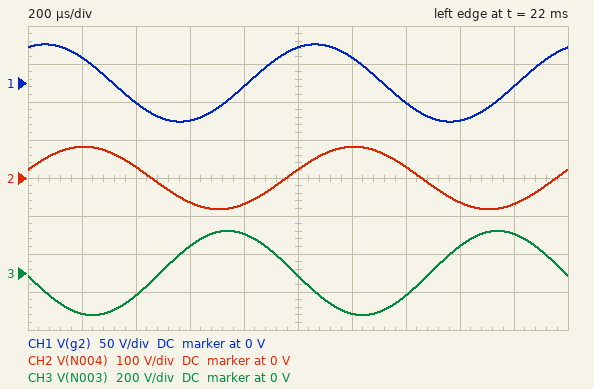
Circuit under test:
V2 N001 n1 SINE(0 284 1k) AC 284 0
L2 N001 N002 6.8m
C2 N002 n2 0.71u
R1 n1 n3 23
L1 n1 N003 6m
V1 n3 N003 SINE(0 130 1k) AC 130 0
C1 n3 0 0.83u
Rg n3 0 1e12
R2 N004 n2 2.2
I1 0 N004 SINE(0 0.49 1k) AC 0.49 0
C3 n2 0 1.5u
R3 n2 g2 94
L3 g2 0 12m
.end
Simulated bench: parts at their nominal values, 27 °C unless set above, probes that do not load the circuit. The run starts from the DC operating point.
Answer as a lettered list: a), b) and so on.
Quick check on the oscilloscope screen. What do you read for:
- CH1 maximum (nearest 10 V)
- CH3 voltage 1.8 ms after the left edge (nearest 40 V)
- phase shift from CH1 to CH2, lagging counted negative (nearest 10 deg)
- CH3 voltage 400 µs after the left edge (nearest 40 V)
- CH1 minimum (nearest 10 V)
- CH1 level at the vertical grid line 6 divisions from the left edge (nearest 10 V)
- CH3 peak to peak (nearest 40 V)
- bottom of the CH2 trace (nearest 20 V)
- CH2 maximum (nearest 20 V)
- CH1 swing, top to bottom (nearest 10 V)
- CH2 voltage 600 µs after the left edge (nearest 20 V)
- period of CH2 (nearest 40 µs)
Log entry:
a) 50 V
b) 200 V
c) -50 deg
d) -120 V
e) -50 V
f) 30 V
g) 440 V
h) -80 V
i) 80 V
j) 100 V
k) -60 V
l) 1.00 ms
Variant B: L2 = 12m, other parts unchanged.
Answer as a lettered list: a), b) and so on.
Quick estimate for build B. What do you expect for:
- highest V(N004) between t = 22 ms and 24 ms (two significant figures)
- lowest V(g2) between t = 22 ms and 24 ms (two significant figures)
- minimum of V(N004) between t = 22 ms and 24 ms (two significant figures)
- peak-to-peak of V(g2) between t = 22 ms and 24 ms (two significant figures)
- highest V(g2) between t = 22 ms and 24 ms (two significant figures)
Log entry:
a) 86 V
b) -53 V
c) -86 V
d) 110 V
e) 53 V
